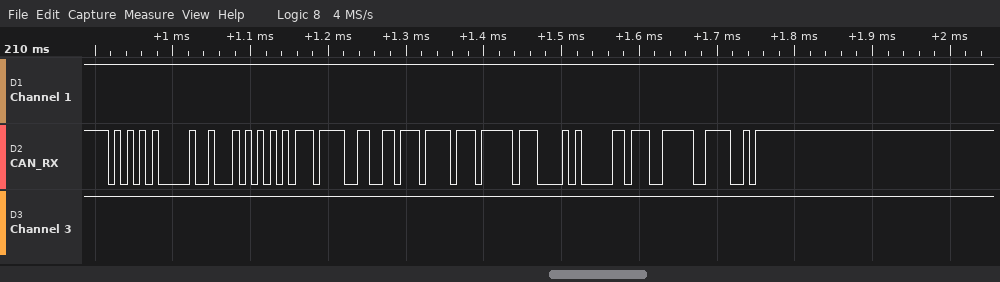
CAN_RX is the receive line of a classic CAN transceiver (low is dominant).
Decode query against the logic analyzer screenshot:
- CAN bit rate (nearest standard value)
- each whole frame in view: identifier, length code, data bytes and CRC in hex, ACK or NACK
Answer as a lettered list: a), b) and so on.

a) 125 kbit/s
b) ID 550, DLC 8, data AA BB CC DD EE FF 0A 0B, CRC 4FBC, ACK
